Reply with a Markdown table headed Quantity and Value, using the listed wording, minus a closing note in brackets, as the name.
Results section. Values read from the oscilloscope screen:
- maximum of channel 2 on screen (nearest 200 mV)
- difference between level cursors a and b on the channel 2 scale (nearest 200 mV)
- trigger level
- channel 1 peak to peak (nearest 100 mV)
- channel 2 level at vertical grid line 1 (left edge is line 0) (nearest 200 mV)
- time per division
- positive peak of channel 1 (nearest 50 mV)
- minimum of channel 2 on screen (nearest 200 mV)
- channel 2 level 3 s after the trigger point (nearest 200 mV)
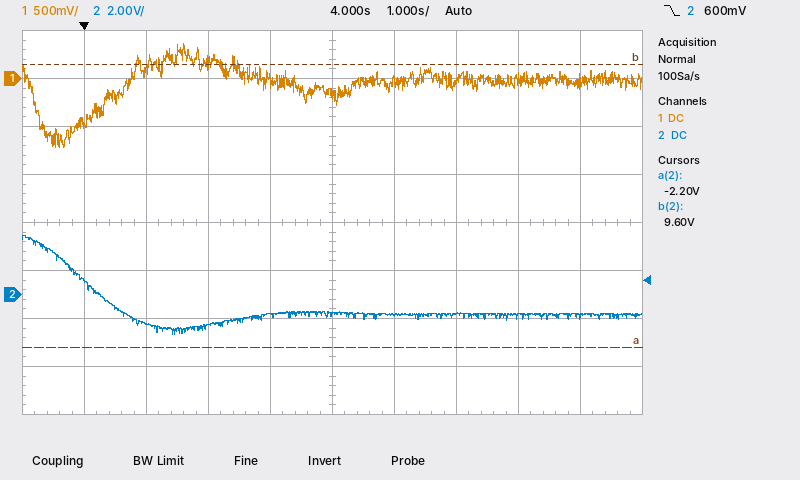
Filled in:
| Quantity | Value |
|---|---|
| maximum of channel 2 on screen | 2.4 V |
| difference between level cursors a and b on the channel 2 scale | 11.8 V |
| trigger level | 600 mV |
| channel 1 peak to peak | 1.10 V |
| channel 2 level at vertical grid line 1 (left edge is line 0) | 600 mV |
| time per division | 1 s |
| positive peak of channel 1 | 350 mV |
| minimum of channel 2 on screen | -1.6 V |
| channel 2 level 3 s after the trigger point | -800 mV |
